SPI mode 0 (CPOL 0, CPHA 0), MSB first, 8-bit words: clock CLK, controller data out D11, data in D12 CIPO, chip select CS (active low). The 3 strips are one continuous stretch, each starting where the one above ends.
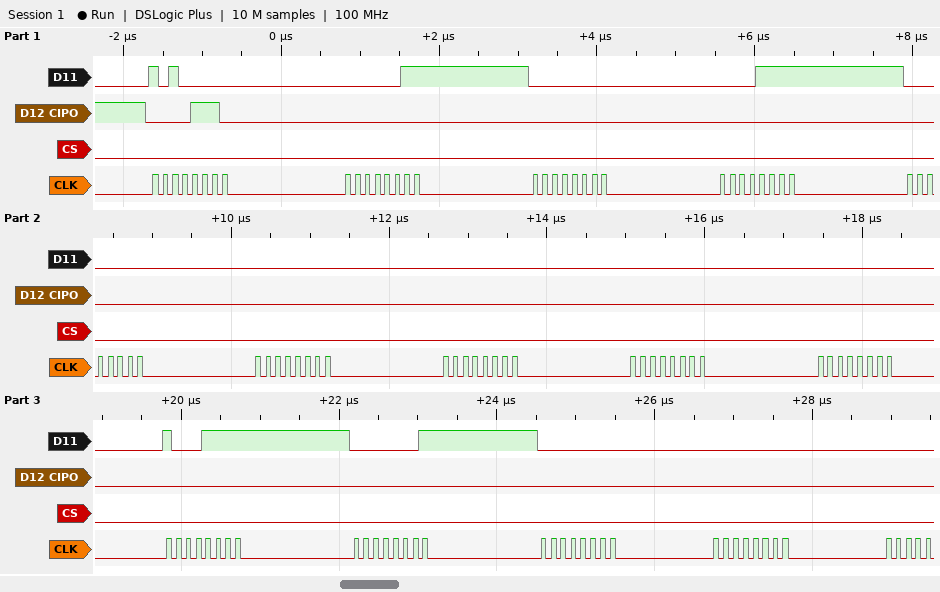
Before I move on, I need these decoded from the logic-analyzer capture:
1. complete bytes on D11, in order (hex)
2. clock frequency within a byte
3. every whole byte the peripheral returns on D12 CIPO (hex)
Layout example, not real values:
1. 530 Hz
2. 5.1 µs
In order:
1. A0 03 00 0F 00 00 00 00 00 8F 01 00 00
2. 8 MHz
3. 0E 00 00 00 00 00 00 00 00 00 00 00 00
